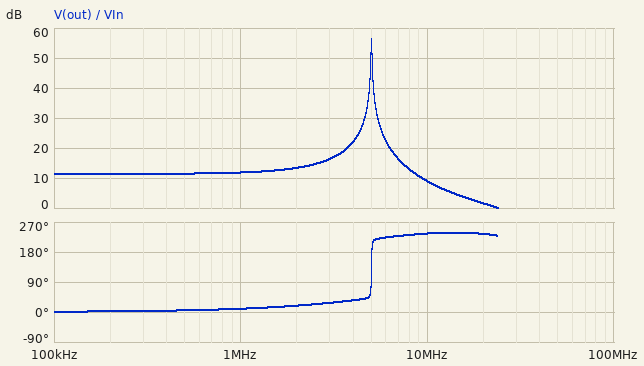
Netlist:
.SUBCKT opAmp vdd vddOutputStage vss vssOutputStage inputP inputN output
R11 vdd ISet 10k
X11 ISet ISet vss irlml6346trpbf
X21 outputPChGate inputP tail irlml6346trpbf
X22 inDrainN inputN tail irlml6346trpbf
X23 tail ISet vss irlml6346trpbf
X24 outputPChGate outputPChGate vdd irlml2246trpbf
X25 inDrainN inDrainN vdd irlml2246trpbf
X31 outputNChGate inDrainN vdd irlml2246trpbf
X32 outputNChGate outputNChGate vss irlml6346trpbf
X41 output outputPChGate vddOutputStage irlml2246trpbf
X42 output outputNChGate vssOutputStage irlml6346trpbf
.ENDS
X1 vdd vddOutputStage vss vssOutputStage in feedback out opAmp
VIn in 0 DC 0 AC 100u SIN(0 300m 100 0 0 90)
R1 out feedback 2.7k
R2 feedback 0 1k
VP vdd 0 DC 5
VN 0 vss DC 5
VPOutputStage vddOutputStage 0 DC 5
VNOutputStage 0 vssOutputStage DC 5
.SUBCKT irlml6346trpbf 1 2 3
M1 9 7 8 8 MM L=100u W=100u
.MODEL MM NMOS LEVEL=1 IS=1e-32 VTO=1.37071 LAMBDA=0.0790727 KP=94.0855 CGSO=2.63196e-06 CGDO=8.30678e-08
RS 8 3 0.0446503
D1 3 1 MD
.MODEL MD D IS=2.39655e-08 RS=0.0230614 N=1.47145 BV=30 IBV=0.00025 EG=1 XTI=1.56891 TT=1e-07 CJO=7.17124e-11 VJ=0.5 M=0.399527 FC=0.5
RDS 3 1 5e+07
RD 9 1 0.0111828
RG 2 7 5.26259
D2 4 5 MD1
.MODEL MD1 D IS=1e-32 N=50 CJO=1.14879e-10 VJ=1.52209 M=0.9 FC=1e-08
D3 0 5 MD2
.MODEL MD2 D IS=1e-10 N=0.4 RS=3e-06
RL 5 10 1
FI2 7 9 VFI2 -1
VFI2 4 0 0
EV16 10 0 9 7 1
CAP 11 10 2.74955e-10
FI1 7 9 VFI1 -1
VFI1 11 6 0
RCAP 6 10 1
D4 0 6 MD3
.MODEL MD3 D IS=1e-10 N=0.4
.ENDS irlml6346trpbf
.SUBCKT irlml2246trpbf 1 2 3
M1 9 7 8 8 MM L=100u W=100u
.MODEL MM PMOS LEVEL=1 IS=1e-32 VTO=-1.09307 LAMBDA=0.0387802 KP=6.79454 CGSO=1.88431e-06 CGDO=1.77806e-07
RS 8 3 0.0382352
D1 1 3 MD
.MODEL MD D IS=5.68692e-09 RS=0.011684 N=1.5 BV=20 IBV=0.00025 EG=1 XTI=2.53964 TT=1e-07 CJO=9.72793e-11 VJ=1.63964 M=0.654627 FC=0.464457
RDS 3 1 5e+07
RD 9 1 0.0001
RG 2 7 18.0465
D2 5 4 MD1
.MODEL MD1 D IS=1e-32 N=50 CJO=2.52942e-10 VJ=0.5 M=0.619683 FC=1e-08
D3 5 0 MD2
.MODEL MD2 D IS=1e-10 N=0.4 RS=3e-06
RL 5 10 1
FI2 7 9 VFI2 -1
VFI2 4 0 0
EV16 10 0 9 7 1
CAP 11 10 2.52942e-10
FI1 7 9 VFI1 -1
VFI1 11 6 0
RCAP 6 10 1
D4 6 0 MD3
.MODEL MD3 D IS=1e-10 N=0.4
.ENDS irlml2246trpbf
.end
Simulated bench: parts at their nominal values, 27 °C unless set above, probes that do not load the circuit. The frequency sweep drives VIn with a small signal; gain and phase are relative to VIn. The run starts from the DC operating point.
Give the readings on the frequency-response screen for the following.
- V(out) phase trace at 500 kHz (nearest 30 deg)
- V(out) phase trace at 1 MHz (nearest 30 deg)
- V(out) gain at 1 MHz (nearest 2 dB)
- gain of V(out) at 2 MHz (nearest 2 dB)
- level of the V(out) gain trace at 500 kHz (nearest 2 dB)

0 deg
0 deg
12 dB
14 dB
12 dB
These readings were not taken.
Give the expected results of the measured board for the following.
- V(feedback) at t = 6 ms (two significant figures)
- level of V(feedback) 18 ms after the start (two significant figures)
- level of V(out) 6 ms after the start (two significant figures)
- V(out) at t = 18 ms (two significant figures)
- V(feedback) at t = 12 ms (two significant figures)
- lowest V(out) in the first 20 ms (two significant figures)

-240 mV
92 mV
-900 mV
340 mV
92 mV
-1.1 V
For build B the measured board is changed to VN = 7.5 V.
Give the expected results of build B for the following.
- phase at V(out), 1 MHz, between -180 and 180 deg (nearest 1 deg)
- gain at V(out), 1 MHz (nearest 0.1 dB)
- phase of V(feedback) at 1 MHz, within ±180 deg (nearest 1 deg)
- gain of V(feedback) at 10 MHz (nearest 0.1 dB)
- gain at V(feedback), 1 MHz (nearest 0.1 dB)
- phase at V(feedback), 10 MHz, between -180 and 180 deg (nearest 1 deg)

-1 deg
12.4 dB
-13 deg
-8.6 dB
0.7 dB
22 deg
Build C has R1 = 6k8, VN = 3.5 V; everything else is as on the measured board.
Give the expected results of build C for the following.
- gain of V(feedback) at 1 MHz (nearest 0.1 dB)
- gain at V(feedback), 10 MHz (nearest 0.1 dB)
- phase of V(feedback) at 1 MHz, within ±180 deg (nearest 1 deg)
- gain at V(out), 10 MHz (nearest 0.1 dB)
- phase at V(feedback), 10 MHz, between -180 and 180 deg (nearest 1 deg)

-2.6 dB
-1.2 dB
31 deg
-53.4 dB
-1 deg
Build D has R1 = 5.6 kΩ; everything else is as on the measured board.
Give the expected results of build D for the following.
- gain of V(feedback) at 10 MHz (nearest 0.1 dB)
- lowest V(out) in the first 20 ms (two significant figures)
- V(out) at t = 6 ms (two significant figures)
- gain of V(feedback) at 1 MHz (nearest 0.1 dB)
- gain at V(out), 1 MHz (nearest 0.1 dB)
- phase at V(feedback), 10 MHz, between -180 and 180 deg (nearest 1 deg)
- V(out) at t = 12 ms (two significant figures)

-1.9 dB
-2.0 V
-1.6 V
0.1 dB
17.3 dB
-1 deg
610 mV
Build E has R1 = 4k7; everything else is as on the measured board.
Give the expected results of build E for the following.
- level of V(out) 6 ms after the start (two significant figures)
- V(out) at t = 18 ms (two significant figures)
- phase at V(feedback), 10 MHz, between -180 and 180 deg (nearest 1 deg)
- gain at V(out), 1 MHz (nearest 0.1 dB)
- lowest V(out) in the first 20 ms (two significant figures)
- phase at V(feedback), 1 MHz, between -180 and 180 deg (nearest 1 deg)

-1.4 V
520 mV
-1 deg
15.9 dB
-1.7 V
-3 deg
